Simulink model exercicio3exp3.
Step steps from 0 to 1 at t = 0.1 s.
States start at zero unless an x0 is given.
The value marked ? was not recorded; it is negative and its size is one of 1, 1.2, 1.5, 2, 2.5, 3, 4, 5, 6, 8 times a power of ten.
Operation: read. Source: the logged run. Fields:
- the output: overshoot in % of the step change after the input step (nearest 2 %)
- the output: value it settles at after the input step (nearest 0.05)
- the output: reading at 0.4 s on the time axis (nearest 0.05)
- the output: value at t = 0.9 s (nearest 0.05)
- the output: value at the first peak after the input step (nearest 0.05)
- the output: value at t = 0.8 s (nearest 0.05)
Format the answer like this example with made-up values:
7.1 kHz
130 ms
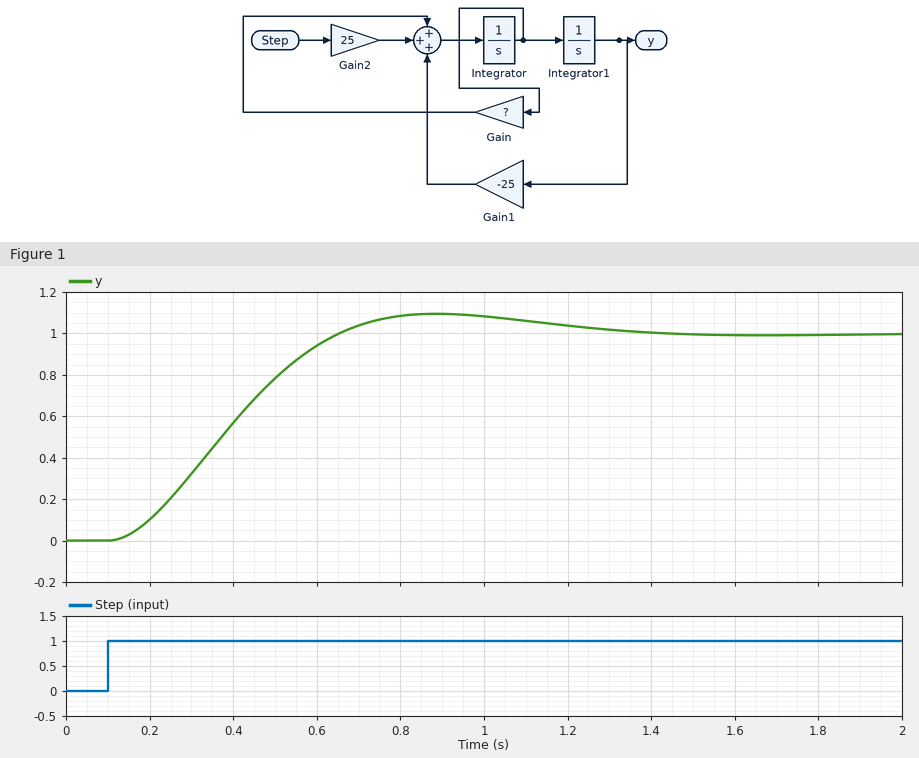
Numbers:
10 %
1.00
0.55
1.10
1.10
1.10
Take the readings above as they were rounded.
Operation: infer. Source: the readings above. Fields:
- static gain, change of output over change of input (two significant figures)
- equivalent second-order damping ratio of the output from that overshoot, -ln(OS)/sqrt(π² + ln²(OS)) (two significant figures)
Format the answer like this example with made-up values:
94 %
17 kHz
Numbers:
1.0
0.59
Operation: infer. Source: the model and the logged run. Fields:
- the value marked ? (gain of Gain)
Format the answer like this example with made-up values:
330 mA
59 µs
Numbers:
-6
